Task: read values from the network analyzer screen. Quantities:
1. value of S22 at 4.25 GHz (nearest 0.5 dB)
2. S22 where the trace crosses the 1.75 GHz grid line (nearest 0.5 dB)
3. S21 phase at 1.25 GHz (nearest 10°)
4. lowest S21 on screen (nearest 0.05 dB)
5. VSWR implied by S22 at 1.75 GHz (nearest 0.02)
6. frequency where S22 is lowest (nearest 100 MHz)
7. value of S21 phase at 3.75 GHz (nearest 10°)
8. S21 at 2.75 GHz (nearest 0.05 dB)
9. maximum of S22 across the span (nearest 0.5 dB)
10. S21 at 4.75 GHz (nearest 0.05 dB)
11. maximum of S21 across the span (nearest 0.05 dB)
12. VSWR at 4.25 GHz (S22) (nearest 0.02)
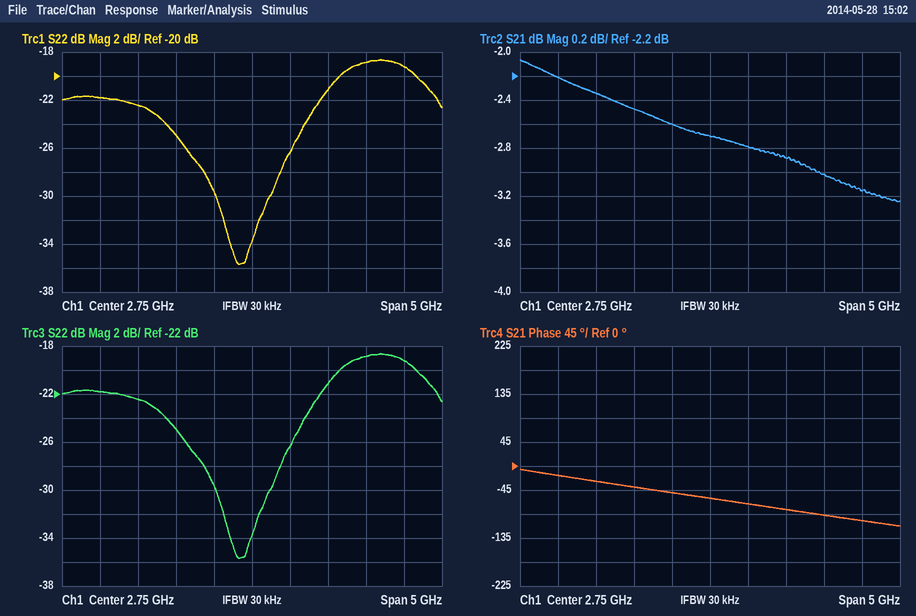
-19.0 dB
-25.0 dB
-30°
-3.25 dB
1.12
2.6 GHz
-80°
-2.70 dB
-18.5 dB
-3.15 dB
-2.05 dB
1.26
